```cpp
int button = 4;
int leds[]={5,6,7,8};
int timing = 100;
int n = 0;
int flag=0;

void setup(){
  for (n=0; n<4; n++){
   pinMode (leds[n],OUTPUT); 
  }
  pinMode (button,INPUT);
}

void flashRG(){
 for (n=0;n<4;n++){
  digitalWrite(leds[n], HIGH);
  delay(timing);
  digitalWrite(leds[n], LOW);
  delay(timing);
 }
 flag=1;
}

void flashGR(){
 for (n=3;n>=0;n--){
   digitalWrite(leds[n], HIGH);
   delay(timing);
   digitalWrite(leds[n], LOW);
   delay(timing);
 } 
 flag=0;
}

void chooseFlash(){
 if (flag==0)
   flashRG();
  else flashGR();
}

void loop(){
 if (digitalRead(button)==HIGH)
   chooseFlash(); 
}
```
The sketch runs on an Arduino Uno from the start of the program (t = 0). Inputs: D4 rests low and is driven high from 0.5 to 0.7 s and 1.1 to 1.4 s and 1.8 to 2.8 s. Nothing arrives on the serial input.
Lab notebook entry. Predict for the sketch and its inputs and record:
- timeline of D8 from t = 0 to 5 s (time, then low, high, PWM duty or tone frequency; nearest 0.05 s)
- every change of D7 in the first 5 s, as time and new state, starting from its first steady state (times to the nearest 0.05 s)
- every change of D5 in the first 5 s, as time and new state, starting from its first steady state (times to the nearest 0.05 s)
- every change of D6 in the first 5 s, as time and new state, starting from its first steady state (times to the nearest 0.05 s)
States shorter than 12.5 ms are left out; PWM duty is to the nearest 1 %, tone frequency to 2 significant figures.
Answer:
0 s low; 1.1 s high; 1.2 s low; 1.3 s high; 1.4 s low; 2.7 s high; 2.8 s low
0 s low; 0.9 s high; 1 s low; 1.5 s high; 1.6 s low; 2.5 s high; 2.6 s low
0 s low; 0.5 s high; 0.6 s low; 1.9 s high; 2 s low; 2.1 s high; 2.2 s low
0 s low; 0.7 s high; 0.8 s low; 1.7 s high; 1.8 s low; 2.3 s high; 2.4 s low
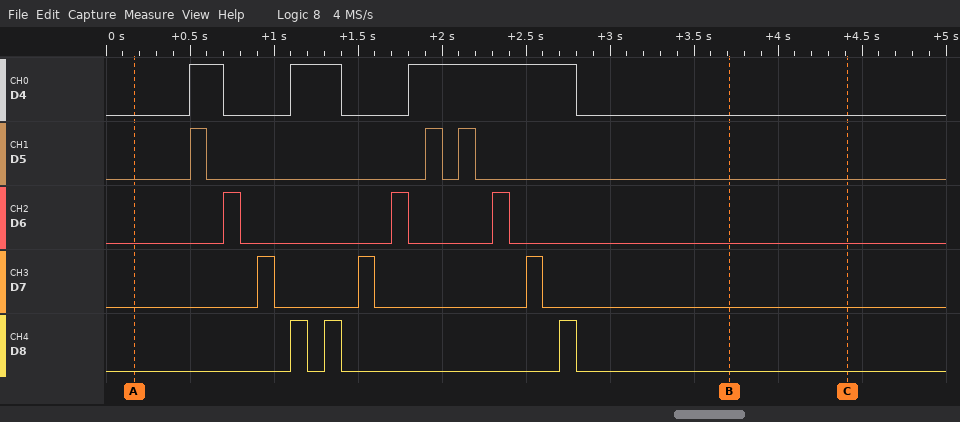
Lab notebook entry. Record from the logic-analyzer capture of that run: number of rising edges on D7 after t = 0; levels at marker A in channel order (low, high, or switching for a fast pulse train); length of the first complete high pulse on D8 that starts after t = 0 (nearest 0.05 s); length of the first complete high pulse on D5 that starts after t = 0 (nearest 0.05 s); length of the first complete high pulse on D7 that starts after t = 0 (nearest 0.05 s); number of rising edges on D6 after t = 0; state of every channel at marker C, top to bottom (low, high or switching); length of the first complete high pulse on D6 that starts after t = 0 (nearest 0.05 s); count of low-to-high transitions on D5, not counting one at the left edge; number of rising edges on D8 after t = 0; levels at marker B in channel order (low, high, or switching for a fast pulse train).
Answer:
3
D4 low, D5 low, D6 low, D7 low, D8 low
0.10 s
0.10 s
0.10 s
3
D4 low, D5 low, D6 low, D7 low, D8 low
0.10 s
3
3
D4 low, D5 low, D6 low, D7 low, D8 low
